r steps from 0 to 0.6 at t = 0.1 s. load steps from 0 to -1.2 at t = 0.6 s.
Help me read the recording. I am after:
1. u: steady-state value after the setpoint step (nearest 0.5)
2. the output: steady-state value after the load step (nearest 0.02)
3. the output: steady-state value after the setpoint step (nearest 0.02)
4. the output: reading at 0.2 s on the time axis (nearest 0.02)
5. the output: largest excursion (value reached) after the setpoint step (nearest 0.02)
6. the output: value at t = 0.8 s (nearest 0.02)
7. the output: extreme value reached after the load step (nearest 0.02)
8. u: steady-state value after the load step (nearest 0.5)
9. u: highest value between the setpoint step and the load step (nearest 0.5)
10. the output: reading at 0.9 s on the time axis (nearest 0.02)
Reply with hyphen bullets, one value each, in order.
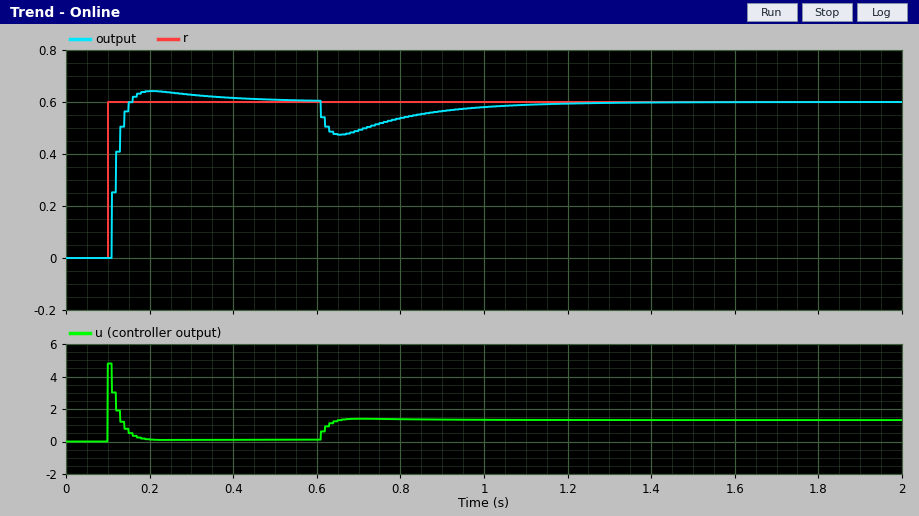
- 0.0
- 0.60
- 0.60
- 0.64
- 0.64
- 0.54
- 0.48
- 1.5
- 5.0
- 0.56
